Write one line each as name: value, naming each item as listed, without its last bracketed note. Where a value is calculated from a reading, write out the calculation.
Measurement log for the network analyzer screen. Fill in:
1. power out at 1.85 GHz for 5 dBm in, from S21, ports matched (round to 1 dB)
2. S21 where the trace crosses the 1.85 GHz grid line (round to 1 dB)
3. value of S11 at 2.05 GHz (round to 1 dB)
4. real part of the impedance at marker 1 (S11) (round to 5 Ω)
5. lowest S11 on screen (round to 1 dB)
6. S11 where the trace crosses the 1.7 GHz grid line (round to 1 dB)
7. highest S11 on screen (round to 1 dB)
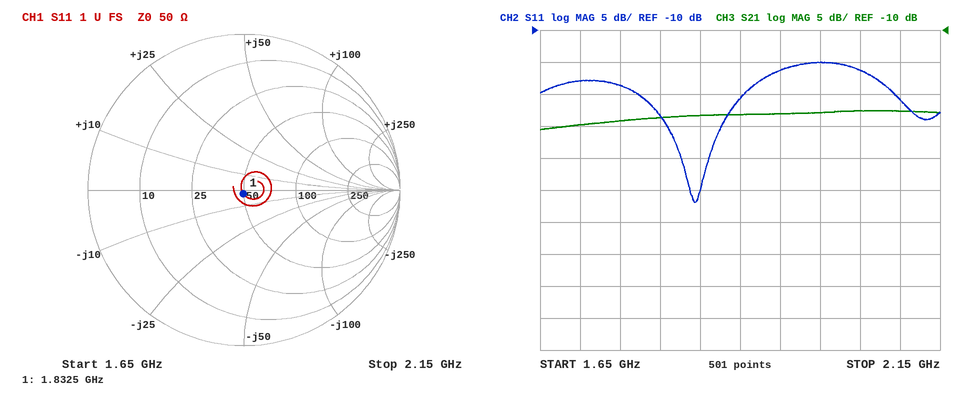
power out at 1.85 GHz for 5 dBm in, from S21, ports matched: 5 dBm + (-23 dB) = -18 dBm
S21 where the trace crosses the 1.85 GHz grid line: -23 dB
value of S11 at 2.05 GHz: -16 dB
real part of the impedance at marker 1 (S11): 50 Ω
lowest S11 on screen: -37 dB
S11 where the trace crosses the 1.7 GHz grid line: -18 dB
highest S11 on screen: -15 dB
